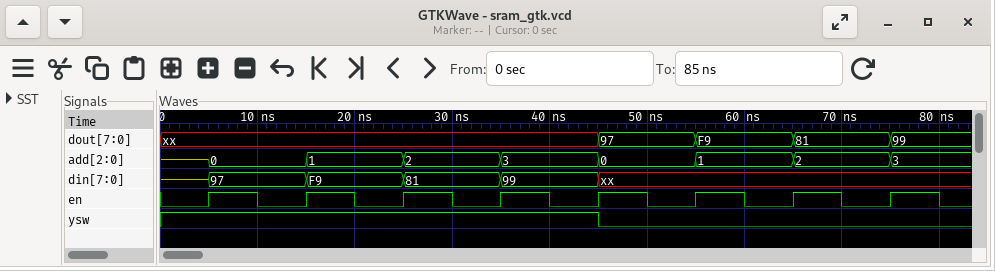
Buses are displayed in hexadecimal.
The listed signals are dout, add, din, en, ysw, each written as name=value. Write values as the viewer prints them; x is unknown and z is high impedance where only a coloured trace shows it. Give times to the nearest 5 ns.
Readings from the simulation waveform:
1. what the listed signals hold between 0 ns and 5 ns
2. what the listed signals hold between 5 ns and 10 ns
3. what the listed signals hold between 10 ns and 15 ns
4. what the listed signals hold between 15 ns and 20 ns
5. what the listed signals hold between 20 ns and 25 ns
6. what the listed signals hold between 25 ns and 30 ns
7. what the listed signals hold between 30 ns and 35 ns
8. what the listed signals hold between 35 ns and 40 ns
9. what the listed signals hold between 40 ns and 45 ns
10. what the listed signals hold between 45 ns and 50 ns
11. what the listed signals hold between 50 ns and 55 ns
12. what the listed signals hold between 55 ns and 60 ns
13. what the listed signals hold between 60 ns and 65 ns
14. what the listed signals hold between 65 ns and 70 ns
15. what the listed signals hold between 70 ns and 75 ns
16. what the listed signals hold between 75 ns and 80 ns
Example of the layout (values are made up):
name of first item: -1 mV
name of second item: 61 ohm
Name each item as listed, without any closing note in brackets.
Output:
what the listed signals hold between 0 ns and 5 ns: dout=xx, add=z, din=z, en=0, ysw=1
what the listed signals hold between 5 ns and 10 ns: dout=xx, add=0, din=97, en=1, ysw=1
what the listed signals hold between 10 ns and 15 ns: dout=xx, add=0, din=97, en=0, ysw=1
what the listed signals hold between 15 ns and 20 ns: dout=xx, add=1, din=F9, en=1, ysw=1
what the listed signals hold between 20 ns and 25 ns: dout=xx, add=1, din=F9, en=0, ysw=1
what the listed signals hold between 25 ns and 30 ns: dout=xx, add=2, din=81, en=1, ysw=1
what the listed signals hold between 30 ns and 35 ns: dout=xx, add=2, din=81, en=0, ysw=1
what the listed signals hold between 35 ns and 40 ns: dout=xx, add=3, din=99, en=1, ysw=1
what the listed signals hold between 40 ns and 45 ns: dout=xx, add=3, din=99, en=0, ysw=1
what the listed signals hold between 45 ns and 50 ns: dout=97, add=0, din=xx, en=1, ysw=0
what the listed signals hold between 50 ns and 55 ns: dout=97, add=0, din=xx, en=0, ysw=0
what the listed signals hold between 55 ns and 60 ns: dout=F9, add=1, din=xx, en=1, ysw=0
what the listed signals hold between 60 ns and 65 ns: dout=F9, add=1, din=xx, en=0, ysw=0
what the listed signals hold between 65 ns and 70 ns: dout=81, add=2, din=xx, en=1, ysw=0
what the listed signals hold between 70 ns and 75 ns: dout=81, add=2, din=xx, en=0, ysw=0
what the listed signals hold between 75 ns and 80 ns: dout=99, add=3, din=xx, en=1, ysw=0
